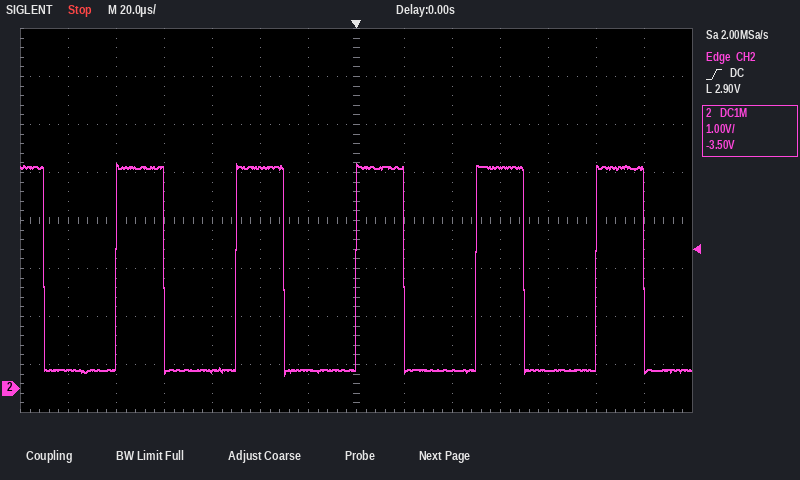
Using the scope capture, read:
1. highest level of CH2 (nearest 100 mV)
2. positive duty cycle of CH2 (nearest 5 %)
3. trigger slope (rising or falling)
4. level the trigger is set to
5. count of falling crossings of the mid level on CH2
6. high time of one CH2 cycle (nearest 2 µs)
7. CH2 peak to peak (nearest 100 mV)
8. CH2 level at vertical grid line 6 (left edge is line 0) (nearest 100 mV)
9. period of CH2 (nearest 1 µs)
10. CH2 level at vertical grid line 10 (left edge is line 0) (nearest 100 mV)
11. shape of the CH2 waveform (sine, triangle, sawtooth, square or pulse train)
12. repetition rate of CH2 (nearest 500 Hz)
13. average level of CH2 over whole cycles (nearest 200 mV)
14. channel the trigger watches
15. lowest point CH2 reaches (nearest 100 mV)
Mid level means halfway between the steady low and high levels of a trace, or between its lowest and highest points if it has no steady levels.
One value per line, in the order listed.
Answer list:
4.7 V
40 %
rising
2.90 V
6
20 µs
4.4 V
400 mV
50 µs
4.6 V
pulse train
20.0 kHz
2.0 V
CH2
300 mV
